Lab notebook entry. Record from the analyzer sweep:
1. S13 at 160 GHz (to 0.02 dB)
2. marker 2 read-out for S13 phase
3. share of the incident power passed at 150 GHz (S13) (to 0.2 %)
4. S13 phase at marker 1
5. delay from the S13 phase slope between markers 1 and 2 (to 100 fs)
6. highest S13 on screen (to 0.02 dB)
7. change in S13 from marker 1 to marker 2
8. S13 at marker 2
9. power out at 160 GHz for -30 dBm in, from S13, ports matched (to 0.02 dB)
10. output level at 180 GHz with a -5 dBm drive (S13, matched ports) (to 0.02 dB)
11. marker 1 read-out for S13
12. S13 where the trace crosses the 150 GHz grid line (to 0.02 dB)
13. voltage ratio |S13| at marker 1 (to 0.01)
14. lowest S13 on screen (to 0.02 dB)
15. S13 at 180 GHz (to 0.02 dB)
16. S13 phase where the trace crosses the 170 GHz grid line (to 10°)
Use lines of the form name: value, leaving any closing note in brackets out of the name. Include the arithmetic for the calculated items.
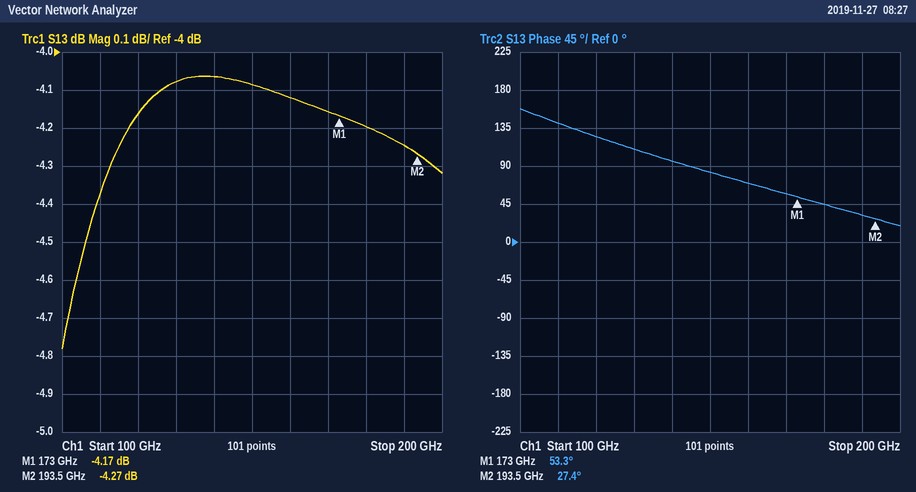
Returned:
S13 at 160 GHz: -4.12 dB
marker 2 read-out for S13 phase: 27.4°
share of the incident power passed at 150 GHz (S13): 10^(-4.08/10) ≈ 39.1 %, so 39.0 % to the nearest 0.2 %
S13 phase at marker 1: 53.3°
delay from the S13 phase slope between markers 1 and 2: −(27.4° − (53.3°))/(360° × 20.5 GHz) ≈ 3.5 ps
highest S13 on screen: -4.06 dB
change in S13 from marker 1 to marker 2: -4.27 − (-4.17) = -0.10 dB
S13 at marker 2: -4.27 dB
power out at 160 GHz for -30 dBm in, from S13, ports matched: -30 dBm + (-4.12 dB) = -34.12 dBm
output level at 180 GHz with a -5 dBm drive (S13, matched ports): -5 dBm + (-4.20 dB) = -9.20 dBm
marker 1 read-out for S13: -4.17 dB
S13 where the trace crosses the 150 GHz grid line: -4.08 dB
voltage ratio |S13| at marker 1: 10^(-4.17/20) ≈ 0.62
lowest S13 on screen: -4.78 dB
S13 at 180 GHz: -4.20 dB
S13 phase where the trace crosses the 170 GHz grid line: 60°
